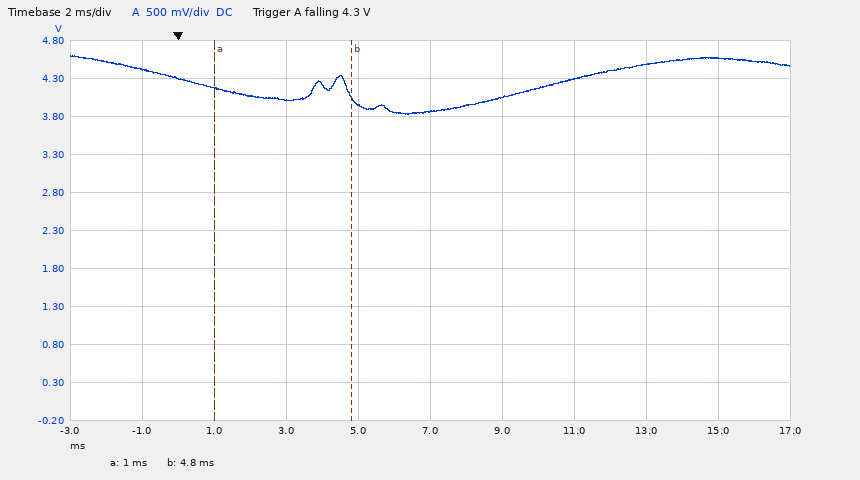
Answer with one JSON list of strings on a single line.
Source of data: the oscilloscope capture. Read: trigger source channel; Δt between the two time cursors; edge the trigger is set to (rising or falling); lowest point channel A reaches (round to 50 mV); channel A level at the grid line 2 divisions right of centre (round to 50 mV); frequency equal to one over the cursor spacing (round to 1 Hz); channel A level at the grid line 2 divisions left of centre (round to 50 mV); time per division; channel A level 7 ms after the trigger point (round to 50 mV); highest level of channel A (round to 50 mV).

["channel A", "3.8 ms", "falling", "3.85 V", "4.30 V", "263 Hz", "4.00 V", "2 ms", "3.85 V", "4.60 V"]
